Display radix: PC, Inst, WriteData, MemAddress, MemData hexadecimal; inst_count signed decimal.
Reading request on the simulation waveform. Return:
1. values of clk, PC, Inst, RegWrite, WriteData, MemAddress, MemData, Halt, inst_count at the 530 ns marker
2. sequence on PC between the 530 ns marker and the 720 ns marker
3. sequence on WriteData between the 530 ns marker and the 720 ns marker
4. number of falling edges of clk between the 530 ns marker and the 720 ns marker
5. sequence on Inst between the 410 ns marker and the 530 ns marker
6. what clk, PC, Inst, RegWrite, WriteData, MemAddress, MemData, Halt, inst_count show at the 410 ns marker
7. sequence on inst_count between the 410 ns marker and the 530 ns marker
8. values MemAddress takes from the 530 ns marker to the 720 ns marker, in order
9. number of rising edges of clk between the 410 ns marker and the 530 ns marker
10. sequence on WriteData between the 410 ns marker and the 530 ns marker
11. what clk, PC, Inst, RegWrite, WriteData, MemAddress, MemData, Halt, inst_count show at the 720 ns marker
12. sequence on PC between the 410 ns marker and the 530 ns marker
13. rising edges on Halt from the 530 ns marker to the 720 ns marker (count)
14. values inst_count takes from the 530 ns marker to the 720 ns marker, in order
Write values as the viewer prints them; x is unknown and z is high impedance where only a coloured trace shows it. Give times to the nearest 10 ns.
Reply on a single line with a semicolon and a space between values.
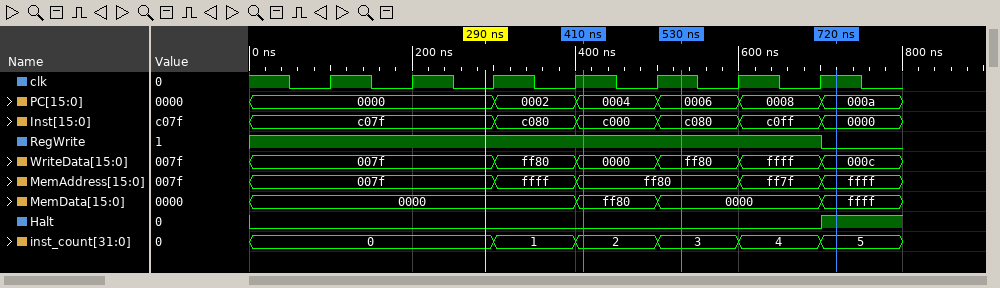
clk=1, PC=0006, Inst=c080, RegWrite=1, WriteData=ff80, MemAddress=ff80, MemData=0000, Halt=0, inst_count=3; 0006, 0008, 000a; ff80, ffff, 000c; 2; c000, c080; clk=1, PC=0004, Inst=c000, RegWrite=1, WriteData=0000, MemAddress=ff80, MemData=ff80, Halt=0, inst_count=2; 2, 3; ff80, ff7f, ffff; 1; 0000, ff80; clk=1, PC=000a, Inst=0000, RegWrite=0, WriteData=000c, MemAddress=ffff, MemData=ffff, Halt=1, inst_count=5; 0004, 0006; 1; 3, 4, 5
